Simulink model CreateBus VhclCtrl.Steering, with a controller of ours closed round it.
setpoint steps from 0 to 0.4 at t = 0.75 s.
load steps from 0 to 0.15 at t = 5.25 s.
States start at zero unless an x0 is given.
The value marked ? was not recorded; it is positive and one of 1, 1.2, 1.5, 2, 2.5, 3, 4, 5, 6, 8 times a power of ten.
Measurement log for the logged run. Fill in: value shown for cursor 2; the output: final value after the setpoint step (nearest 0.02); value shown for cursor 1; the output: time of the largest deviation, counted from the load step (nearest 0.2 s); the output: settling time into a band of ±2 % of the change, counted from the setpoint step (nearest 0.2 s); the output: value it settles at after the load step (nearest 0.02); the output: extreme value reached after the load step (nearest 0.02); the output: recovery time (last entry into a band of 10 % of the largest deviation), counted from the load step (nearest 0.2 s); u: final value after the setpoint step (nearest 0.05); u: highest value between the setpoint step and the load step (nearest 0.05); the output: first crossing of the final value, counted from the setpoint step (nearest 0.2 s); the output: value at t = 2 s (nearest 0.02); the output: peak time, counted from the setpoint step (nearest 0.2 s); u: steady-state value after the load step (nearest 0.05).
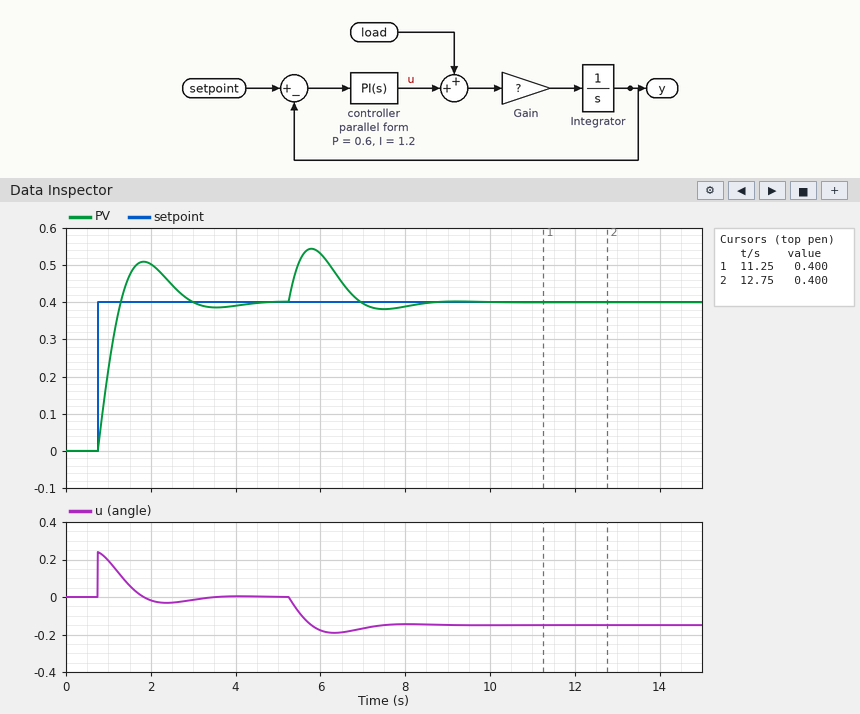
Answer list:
0.400
0.40
0.400
0.6 s
3.4 s
0.40
0.54
2.6 s
0.00
0.25
0.6 s
0.50
1.0 s
-0.15
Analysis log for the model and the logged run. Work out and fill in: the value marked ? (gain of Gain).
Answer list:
4
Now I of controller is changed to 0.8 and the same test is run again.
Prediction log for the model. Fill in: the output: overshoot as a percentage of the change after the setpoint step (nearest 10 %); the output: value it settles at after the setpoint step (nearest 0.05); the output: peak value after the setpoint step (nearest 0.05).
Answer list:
20 %
0.40
0.50
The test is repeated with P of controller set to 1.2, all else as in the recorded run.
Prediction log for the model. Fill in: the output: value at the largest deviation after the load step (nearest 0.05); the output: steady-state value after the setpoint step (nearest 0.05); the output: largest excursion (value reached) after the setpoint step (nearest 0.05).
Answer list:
0.50
0.40
0.45
